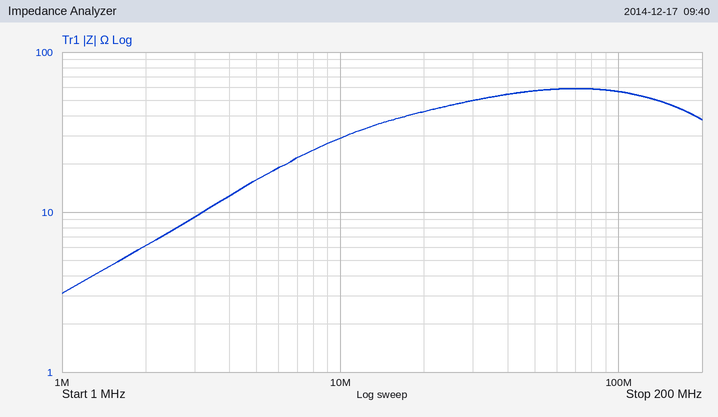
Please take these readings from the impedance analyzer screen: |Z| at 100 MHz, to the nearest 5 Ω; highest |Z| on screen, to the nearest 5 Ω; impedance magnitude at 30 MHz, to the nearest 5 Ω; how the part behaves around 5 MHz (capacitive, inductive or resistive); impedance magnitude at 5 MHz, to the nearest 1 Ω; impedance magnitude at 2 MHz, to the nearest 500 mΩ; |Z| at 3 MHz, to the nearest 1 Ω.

55 Ω
60 Ω
50 Ω
inductive
16 Ω
6.0 Ω
9 Ω
